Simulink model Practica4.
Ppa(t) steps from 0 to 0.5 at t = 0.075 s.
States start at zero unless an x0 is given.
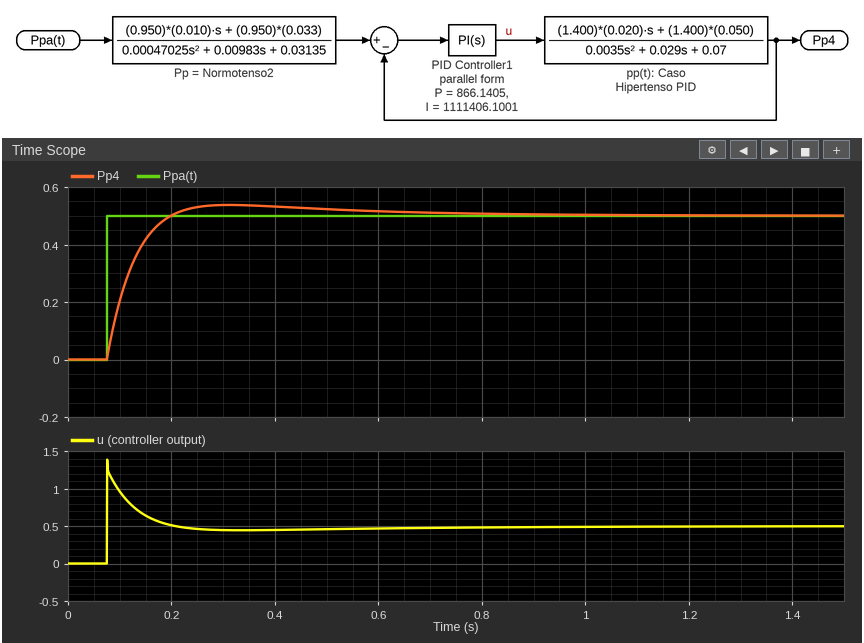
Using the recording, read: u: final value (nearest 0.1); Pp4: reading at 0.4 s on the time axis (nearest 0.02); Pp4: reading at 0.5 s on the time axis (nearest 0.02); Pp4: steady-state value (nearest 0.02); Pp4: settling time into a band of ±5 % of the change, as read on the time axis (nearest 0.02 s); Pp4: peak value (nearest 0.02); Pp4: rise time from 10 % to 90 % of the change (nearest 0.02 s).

0.5
0.54
0.52
0.50
0.48 s
0.54
0.08 s
